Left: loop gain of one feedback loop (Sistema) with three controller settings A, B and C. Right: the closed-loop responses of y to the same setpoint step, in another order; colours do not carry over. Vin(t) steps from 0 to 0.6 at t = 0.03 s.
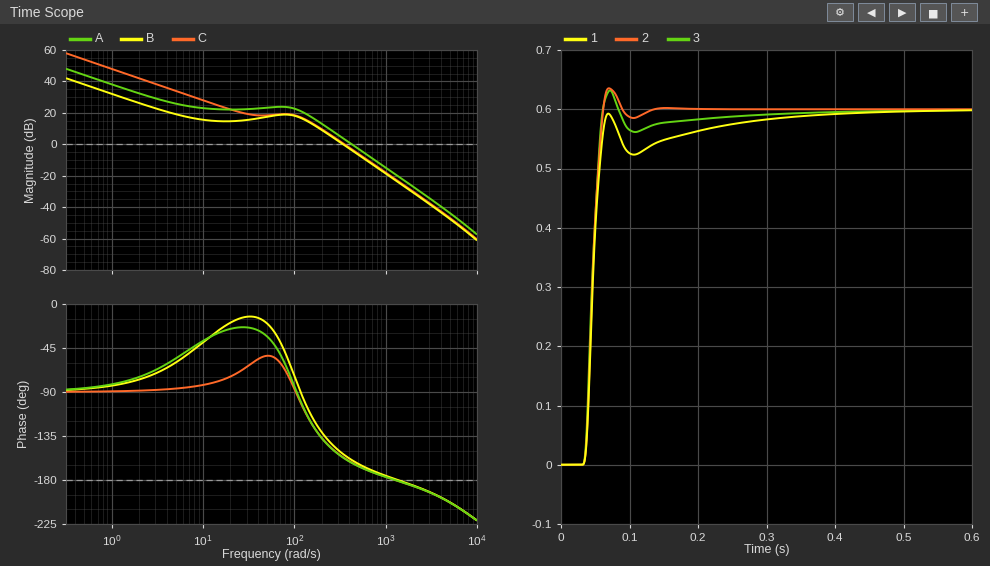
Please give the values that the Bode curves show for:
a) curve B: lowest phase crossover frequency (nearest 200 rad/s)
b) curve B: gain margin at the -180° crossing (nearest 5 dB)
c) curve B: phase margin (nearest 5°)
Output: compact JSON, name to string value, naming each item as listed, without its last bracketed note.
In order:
{"curve B: lowest phase crossover frequency": "1400 rad/s", "curve B: gain margin at the -180° crossing": "25 dB", "curve B: phase margin": "25°"}
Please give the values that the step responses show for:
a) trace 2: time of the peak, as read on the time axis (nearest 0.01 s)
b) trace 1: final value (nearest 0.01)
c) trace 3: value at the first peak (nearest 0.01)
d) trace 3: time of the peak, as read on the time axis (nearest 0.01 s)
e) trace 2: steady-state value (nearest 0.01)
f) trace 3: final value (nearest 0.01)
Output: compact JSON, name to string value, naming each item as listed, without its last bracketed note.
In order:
{"trace 2: time of the peak, as read on the time axis": "0.07 s", "trace 1: final value": "0.60", "trace 3: value at the first peak": "0.63", "trace 3: time of the peak, as read on the time axis": "0.07 s", "trace 2: steady-state value": "0.60", "trace 3: final value": "0.60"}
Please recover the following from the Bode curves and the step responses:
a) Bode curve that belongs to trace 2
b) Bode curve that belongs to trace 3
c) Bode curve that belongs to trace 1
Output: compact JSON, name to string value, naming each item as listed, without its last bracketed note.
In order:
{"Bode curve that belongs to trace 2": "C", "Bode curve that belongs to trace 3": "A", "Bode curve that belongs to trace 1": "B"}
